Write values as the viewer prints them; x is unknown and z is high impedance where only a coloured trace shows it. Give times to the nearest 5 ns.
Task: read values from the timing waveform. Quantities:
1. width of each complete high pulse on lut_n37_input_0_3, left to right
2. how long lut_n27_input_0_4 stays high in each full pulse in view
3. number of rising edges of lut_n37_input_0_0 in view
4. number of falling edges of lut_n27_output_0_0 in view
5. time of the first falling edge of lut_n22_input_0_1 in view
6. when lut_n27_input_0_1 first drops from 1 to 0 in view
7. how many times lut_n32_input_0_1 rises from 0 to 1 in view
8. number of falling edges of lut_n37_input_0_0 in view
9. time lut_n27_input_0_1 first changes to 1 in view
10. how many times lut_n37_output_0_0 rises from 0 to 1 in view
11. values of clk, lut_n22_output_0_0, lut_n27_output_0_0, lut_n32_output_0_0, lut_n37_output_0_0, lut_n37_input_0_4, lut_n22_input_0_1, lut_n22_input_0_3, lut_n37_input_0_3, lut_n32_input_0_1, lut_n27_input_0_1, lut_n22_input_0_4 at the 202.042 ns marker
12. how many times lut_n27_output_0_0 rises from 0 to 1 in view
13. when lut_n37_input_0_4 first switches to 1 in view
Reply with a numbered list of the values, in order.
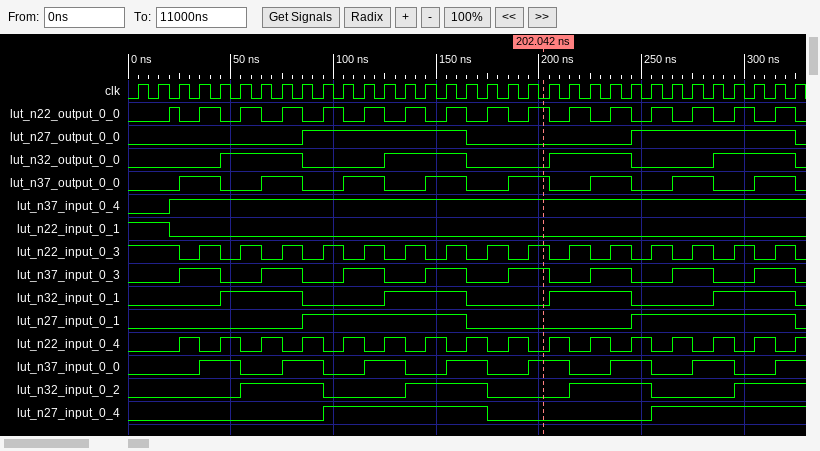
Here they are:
1. 20 ns, 20 ns, 20 ns, 20 ns, 20 ns, 20 ns, 20 ns, 20 ns
2. 80 ns
3. 8
4. 2
5. 20 ns
6. 165 ns
7. 4
8. 7
9. 85 ns
10. 8
11. clk=0, lut_n22_output_0_0=1, lut_n27_output_0_0=0, lut_n32_output_0_0=0, lut_n37_output_0_0=1, lut_n37_input_0_4=1, lut_n22_input_0_1=0, lut_n22_input_0_3=1, lut_n37_input_0_3=1, lut_n32_input_0_1=0, lut_n27_input_0_1=0, lut_n22_input_0_4=0
12. 2
13. 20 ns
